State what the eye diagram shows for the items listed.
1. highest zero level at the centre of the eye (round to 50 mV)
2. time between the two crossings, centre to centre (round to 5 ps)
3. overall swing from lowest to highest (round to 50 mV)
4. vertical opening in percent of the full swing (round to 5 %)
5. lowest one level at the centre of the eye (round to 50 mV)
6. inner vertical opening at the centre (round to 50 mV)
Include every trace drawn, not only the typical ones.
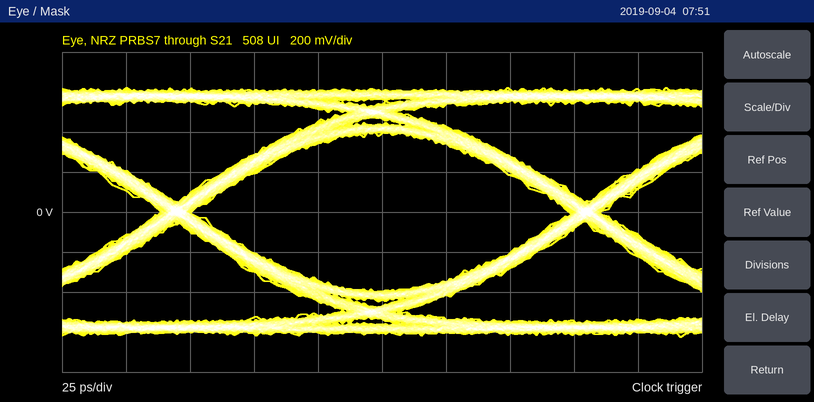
-400 mV
160 ps
1.25 V
65 %
400 mV
800 mV
